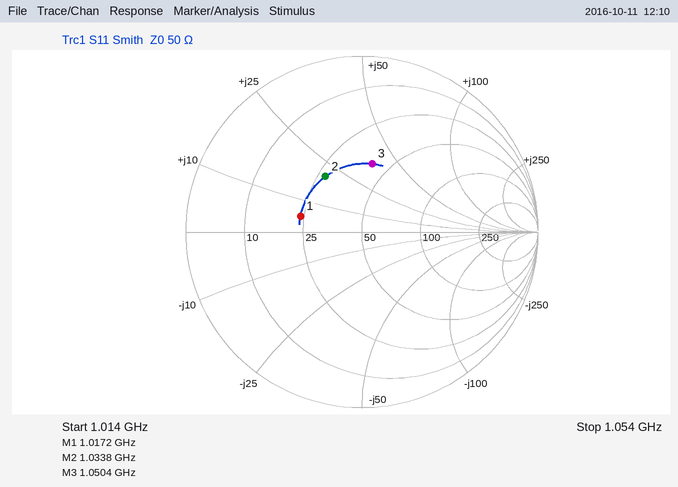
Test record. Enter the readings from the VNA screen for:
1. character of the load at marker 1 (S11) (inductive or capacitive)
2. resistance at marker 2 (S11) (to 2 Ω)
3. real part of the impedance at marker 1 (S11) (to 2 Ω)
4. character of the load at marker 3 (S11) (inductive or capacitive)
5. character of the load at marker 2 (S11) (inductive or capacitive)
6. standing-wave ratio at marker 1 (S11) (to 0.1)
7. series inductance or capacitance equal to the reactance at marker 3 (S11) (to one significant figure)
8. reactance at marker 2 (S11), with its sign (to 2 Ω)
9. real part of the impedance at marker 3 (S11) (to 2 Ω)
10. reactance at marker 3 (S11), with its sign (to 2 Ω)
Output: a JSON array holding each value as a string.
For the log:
["inductive", "28 Ω", "24 Ω", "inductive", "inductive", "2.1", "6 nH", "+20 Ω", "40 Ω", "+38 Ω"]
